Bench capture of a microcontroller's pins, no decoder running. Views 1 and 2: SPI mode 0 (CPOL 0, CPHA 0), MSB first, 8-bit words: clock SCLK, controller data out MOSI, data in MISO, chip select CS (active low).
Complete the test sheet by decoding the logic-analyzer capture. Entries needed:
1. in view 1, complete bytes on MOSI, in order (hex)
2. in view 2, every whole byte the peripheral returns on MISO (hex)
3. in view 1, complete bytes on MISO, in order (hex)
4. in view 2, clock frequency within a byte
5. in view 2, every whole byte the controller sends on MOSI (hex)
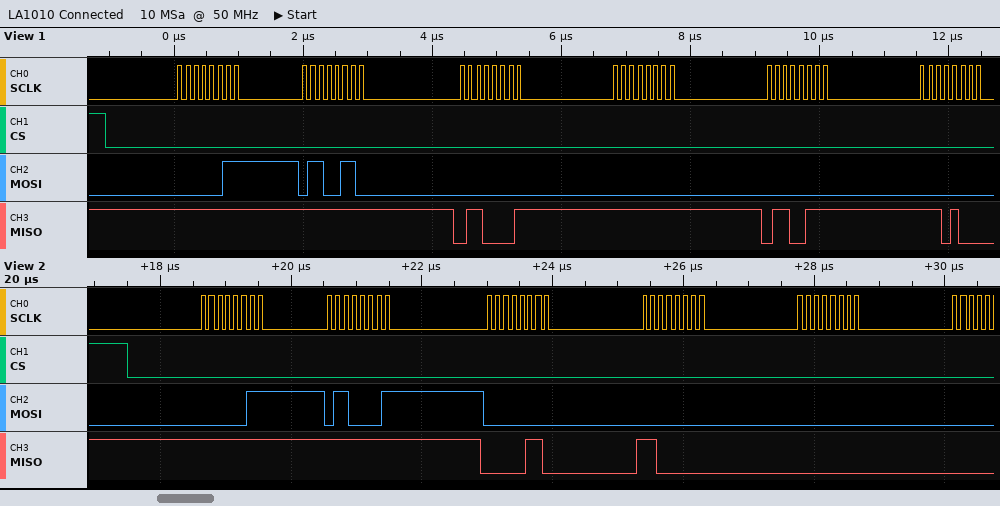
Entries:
03 66 00 00 00 00
FF FF 06 C0 00
FF FF 61 FF 67 E8
8 MHz
03 61 00 00 00
